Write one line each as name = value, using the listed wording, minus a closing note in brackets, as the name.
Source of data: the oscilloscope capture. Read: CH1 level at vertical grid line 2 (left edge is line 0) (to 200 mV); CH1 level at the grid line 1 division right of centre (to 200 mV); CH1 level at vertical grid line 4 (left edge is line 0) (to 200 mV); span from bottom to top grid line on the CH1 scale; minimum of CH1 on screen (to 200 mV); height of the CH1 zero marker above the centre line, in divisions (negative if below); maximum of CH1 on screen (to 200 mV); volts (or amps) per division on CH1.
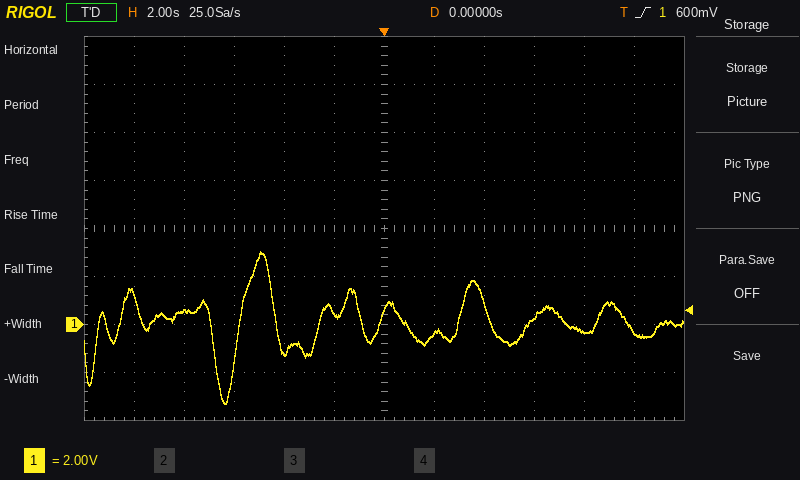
CH1 level at vertical grid line 2 (left edge is line 0) = 600 mV
CH1 level at the grid line 1 division right of centre = -400 mV
CH1 level at vertical grid line 4 (left edge is line 0) = -1.2 V
span from bottom to top grid line on the CH1 scale = 16 V
minimum of CH1 on screen = -3.2 V
height of the CH1 zero marker above the centre line, in divisions = -2.0 div
maximum of CH1 on screen = 3.0 V
volts (or amps) per division on CH1 = 2 V
